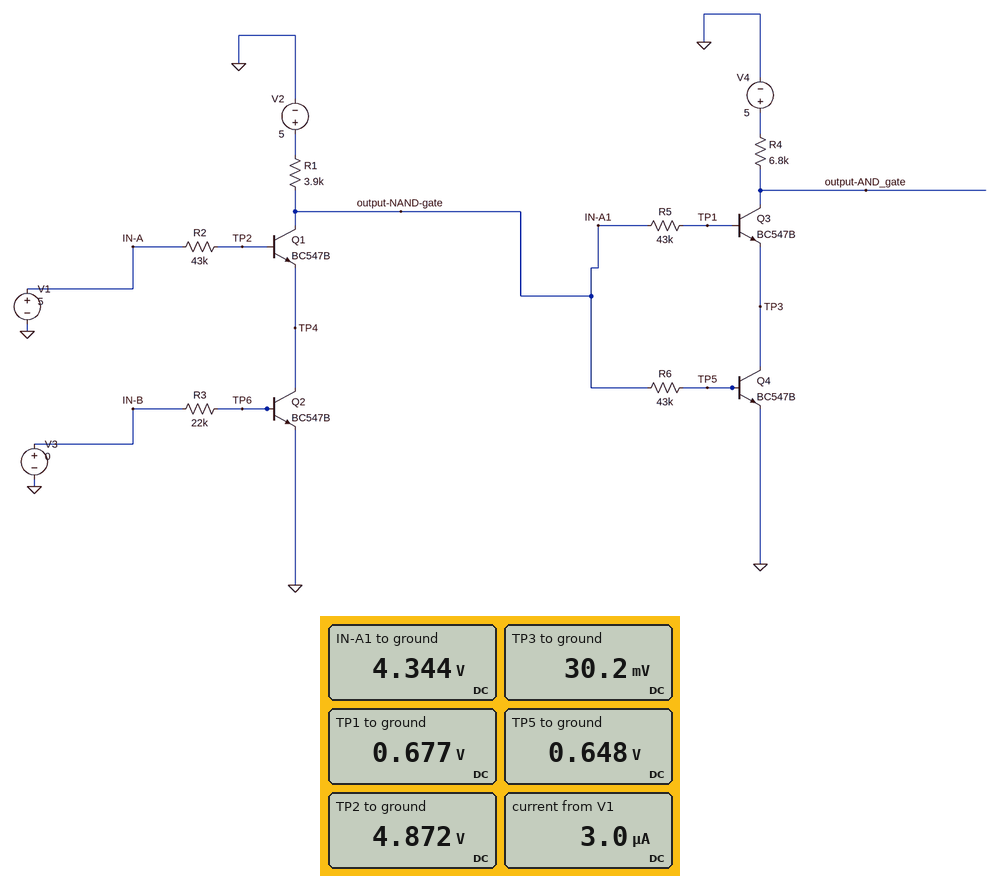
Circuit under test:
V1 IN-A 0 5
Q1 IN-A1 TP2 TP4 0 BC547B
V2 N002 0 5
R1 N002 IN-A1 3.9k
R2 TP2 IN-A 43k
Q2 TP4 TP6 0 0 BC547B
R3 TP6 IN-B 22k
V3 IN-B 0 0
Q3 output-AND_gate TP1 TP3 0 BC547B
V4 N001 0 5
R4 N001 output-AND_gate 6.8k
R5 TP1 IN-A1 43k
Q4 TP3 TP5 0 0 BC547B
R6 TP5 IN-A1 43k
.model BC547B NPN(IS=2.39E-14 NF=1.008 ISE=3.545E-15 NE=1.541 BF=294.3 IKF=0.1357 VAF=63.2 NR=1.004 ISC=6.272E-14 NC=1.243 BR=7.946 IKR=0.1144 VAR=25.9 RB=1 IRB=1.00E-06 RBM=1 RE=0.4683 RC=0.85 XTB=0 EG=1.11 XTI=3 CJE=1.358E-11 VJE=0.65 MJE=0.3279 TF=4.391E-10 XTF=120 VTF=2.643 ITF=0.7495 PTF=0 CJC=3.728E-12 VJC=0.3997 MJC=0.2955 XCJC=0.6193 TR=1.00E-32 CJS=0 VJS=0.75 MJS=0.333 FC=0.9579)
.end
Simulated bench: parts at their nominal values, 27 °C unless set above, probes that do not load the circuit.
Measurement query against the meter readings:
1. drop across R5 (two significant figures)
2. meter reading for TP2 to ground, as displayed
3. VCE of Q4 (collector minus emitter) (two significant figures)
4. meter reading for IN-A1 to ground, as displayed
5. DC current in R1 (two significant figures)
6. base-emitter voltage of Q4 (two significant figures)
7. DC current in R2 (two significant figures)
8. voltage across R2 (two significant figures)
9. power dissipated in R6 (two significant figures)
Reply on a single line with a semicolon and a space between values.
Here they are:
3.7 V; 4.872 V; 30 mV; 4.344 V; 170 µA; 650 mV; 3.0 µA; 130 mV; 320 µW
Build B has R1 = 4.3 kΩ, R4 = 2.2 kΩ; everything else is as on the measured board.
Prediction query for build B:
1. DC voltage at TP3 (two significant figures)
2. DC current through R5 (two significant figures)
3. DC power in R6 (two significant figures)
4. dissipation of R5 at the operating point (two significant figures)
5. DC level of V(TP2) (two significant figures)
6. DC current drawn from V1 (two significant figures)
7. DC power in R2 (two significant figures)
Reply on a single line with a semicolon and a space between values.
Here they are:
53 mV; 83 µA; 310 µW; 300 µW; 4.8 V; 3.9 µA; 660 nW
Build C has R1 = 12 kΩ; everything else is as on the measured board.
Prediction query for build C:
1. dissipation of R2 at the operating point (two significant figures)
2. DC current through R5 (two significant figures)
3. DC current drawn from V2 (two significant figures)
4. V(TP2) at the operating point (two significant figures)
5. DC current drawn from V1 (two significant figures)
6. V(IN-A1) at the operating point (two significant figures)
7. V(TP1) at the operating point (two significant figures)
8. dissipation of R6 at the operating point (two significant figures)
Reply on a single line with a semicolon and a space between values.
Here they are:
16 µW; 68 µA; 120 µA; 4.2 V; 19 µA; 3.6 V; 680 mV; 200 µW
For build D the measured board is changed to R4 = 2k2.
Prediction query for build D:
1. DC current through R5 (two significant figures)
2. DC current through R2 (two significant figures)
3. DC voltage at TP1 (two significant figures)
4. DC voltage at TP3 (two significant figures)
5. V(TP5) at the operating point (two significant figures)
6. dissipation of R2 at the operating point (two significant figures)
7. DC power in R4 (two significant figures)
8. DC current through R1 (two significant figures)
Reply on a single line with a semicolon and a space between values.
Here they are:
84 µA; 2.9 µA; 720 mV; 53 mV; 670 mV; 360 nW; 11 mW; 170 µA
